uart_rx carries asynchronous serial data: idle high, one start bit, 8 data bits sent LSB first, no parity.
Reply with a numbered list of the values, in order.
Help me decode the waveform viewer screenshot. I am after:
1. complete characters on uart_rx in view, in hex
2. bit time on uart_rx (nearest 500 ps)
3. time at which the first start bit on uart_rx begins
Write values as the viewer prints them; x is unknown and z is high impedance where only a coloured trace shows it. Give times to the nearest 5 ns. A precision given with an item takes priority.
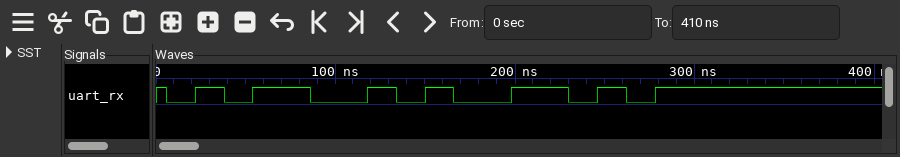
1. 4D, D6
2. 16000 ps
3. 5 ns
